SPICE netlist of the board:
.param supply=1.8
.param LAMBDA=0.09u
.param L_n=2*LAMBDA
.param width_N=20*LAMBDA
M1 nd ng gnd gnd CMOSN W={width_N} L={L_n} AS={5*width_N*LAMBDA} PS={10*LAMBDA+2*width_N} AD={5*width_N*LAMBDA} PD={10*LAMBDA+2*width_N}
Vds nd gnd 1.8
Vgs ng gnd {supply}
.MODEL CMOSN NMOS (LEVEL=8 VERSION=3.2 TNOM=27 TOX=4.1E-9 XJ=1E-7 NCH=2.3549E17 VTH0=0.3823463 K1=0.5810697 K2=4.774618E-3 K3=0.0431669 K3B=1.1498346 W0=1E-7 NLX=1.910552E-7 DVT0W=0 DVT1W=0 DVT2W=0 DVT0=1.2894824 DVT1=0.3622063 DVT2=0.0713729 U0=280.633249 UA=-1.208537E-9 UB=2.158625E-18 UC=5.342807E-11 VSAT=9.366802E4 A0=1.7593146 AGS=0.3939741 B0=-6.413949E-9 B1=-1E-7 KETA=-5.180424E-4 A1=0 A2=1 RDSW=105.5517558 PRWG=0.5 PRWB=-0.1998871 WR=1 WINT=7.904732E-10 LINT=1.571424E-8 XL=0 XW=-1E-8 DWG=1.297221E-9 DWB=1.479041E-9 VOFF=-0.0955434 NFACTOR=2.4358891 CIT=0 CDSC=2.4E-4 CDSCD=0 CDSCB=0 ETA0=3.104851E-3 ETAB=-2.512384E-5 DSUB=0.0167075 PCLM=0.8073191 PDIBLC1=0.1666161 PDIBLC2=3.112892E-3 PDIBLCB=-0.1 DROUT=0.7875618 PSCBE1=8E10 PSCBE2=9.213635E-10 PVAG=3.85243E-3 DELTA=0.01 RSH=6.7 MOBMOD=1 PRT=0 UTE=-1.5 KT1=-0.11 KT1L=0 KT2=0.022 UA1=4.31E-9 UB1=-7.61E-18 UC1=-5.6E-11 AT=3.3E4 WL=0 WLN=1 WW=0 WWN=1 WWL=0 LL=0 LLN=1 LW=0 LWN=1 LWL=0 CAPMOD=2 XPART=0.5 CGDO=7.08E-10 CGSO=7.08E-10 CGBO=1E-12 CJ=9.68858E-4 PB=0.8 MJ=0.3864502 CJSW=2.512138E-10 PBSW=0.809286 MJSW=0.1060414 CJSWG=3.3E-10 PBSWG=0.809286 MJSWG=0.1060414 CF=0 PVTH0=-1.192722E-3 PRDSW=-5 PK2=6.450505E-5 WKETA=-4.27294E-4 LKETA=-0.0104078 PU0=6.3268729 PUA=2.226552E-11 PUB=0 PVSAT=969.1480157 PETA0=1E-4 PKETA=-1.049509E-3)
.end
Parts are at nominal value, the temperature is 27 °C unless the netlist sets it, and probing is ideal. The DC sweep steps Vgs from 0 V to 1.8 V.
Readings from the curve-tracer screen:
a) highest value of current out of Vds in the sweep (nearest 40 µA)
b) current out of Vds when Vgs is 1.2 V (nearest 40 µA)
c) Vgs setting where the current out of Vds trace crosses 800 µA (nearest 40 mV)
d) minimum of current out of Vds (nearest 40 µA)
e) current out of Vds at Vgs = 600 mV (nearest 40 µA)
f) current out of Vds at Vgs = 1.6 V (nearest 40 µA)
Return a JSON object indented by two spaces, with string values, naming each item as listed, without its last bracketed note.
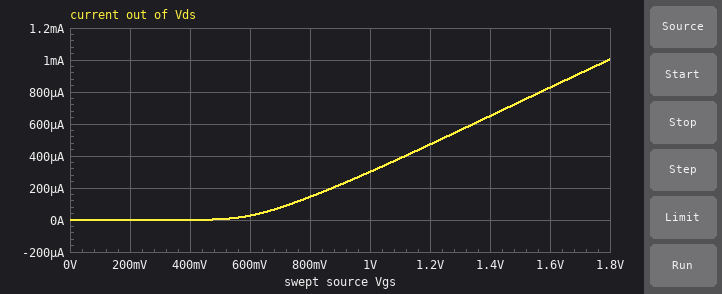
{
  "highest value of current out of Vds in the sweep": "1.00 mA",
  "current out of Vds when Vgs is 1.2 V": "480 µA",
  "Vgs setting where the current out of Vds trace crosses 800 µA": "1.56 V",
  "minimum of current out of Vds": "0 A",
  "current out of Vds at Vgs = 600 mV": "40 µA",
  "current out of Vds at Vgs = 1.6 V": "840 µA"
}
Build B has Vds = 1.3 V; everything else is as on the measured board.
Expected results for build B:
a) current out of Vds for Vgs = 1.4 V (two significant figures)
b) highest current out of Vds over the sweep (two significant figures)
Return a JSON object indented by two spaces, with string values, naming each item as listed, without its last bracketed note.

{
  "current out of Vds for Vgs = 1.4 V": "630 µA",
  "highest current out of Vds over the sweep": "980 µA"
}
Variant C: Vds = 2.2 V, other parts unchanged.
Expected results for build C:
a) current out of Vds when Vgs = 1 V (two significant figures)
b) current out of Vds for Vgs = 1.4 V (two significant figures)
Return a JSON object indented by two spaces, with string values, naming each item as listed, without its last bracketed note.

{
  "current out of Vds when Vgs = 1 V": "310 µA",
  "current out of Vds for Vgs = 1.4 V": "670 µA"
}
